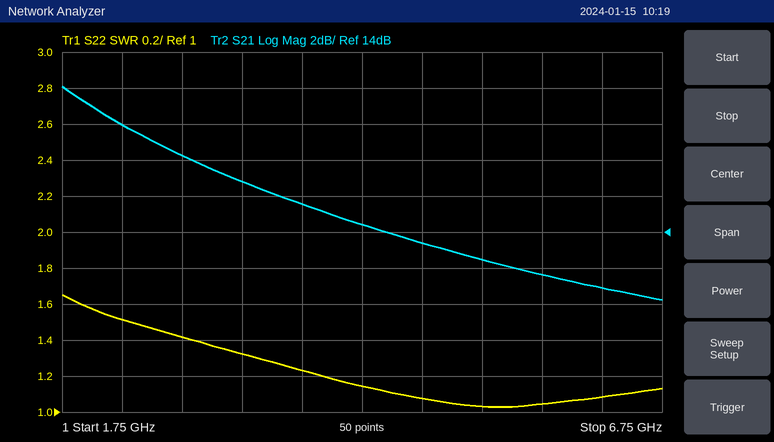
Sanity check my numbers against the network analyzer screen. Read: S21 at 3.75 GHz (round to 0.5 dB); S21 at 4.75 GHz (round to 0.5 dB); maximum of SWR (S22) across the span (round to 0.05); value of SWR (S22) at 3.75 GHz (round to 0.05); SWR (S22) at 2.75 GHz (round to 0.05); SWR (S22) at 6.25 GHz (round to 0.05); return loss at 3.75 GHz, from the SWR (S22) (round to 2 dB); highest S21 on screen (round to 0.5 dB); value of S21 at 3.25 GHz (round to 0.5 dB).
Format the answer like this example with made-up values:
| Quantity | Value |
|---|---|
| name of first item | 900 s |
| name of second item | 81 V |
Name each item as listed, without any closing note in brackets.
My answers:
| Quantity | Value |
|---|---|
| S21 at 3.75 GHz | 15.5 dB |
| S21 at 4.75 GHz | 13.5 dB |
| maximum of SWR (S22) across the span | 1.65 |
| value of SWR (S22) at 3.75 GHz | 1.25 |
| SWR (S22) at 2.75 GHz | 1.40 |
| SWR (S22) at 6.25 GHz | 1.10 |
| return loss at 3.75 GHz, from the SWR (S22) | 20 dB |
| highest S21 on screen | 22.0 dB |
| value of S21 at 3.25 GHz | 17.0 dB |
